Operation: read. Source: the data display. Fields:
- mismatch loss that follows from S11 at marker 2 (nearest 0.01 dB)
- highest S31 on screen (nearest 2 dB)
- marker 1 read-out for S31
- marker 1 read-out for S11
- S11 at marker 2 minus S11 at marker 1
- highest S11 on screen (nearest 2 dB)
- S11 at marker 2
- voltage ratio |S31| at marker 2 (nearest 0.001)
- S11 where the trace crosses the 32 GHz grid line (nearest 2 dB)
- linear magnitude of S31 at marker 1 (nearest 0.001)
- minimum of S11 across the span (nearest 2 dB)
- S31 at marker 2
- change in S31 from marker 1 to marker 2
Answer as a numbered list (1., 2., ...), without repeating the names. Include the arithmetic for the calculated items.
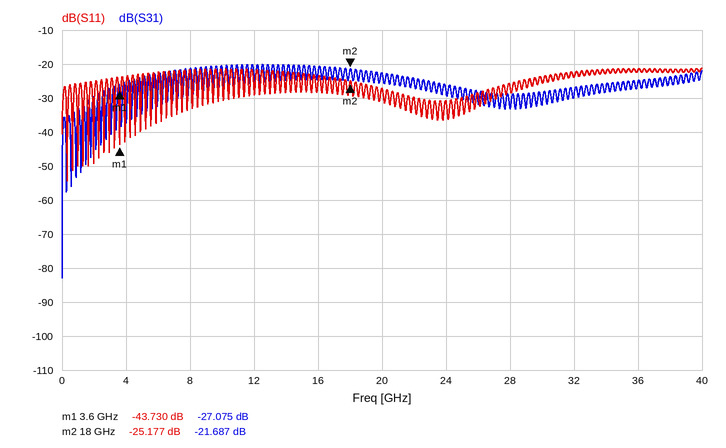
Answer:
1. −10 log10(1 − 10^(-25.177/10)) ≈ 0.01 dB
2. -20 dB
3. -27.075 dB
4. -43.730 dB
5. -25.177 − (-43.73) = 18.553 dB
6. -22 dB
7. -25.177 dB
8. 10^(-21.687/20) ≈ 0.082
9. -24 dB
10. 10^(-27.075/20) ≈ 0.044
11. -54 dB
12. -21.687 dB
13. -21.687 − (-27.075) = 5.388 dB
